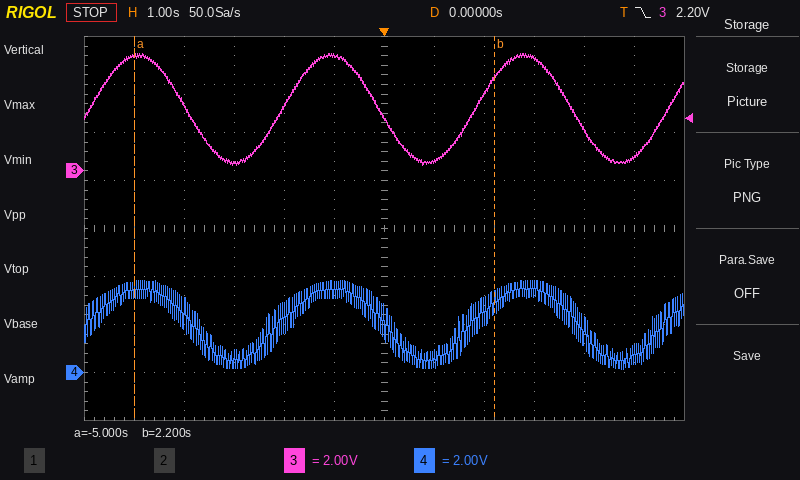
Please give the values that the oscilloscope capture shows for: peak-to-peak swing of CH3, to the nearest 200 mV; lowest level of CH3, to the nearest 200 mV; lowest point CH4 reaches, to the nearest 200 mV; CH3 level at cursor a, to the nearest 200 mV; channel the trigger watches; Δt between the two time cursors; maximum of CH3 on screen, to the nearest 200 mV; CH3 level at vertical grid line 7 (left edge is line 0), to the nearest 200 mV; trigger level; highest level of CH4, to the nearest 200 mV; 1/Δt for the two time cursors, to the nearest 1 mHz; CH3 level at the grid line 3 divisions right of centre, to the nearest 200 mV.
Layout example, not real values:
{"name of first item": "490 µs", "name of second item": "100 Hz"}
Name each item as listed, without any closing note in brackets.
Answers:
{"peak-to-peak swing of CH3, to the nearest 200 mV": "4.6 V", "lowest level of CH3, to the nearest 200 mV": "200 mV", "lowest point CH4 reaches, to the nearest 200 mV": "200 mV", "CH3 level at cursor a, to the nearest 200 mV": "4.8 V", "channel the trigger watches": "CH3", "Δt between the two time cursors": "7.2 s", "maximum of CH3 on screen, to the nearest 200 mV": "4.8 V", "CH3 level at vertical grid line 7 (left edge is line 0), to the nearest 200 mV": "400 mV", "trigger level": "2.20 V", "highest level of CH4, to the nearest 200 mV": "3.8 V", "1/Δt for the two time cursors, to the nearest 1 mHz": "139 mHz", "CH3 level at the grid line 3 divisions right of centre, to the nearest 200 mV": "4.6 V"}
